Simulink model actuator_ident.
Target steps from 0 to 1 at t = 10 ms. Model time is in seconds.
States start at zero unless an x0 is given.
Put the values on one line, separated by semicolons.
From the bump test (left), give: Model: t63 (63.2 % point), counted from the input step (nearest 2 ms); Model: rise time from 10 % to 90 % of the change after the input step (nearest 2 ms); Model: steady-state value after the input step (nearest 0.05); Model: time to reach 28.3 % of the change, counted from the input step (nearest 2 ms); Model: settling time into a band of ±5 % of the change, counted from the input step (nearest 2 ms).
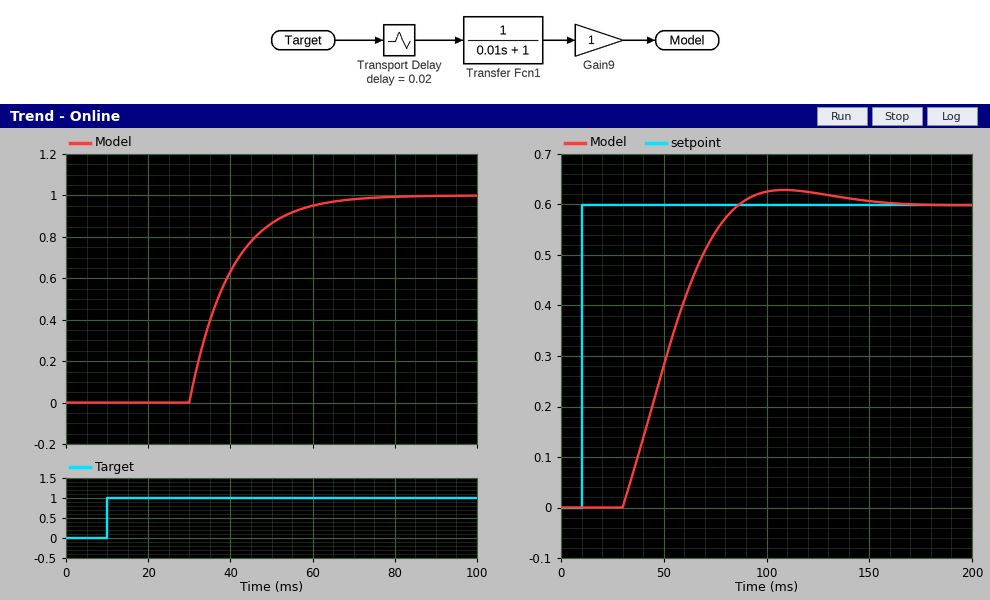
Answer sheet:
30 ms; 22 ms; 1.00; 24 ms; 50 ms
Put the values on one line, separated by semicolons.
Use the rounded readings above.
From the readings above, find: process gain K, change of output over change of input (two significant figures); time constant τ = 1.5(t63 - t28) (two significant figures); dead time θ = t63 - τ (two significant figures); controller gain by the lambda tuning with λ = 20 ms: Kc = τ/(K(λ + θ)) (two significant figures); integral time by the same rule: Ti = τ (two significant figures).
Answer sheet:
1.0; 9.0 ms; 21 ms; 0.22; 9.0 ms
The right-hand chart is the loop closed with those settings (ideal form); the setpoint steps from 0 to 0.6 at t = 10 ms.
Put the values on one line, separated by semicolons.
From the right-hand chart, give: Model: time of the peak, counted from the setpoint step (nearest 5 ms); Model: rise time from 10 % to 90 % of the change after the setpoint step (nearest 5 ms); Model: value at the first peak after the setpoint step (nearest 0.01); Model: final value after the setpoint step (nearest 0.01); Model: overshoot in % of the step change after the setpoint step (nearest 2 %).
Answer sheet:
100 ms; 40 ms; 0.63; 0.60; 4 %
